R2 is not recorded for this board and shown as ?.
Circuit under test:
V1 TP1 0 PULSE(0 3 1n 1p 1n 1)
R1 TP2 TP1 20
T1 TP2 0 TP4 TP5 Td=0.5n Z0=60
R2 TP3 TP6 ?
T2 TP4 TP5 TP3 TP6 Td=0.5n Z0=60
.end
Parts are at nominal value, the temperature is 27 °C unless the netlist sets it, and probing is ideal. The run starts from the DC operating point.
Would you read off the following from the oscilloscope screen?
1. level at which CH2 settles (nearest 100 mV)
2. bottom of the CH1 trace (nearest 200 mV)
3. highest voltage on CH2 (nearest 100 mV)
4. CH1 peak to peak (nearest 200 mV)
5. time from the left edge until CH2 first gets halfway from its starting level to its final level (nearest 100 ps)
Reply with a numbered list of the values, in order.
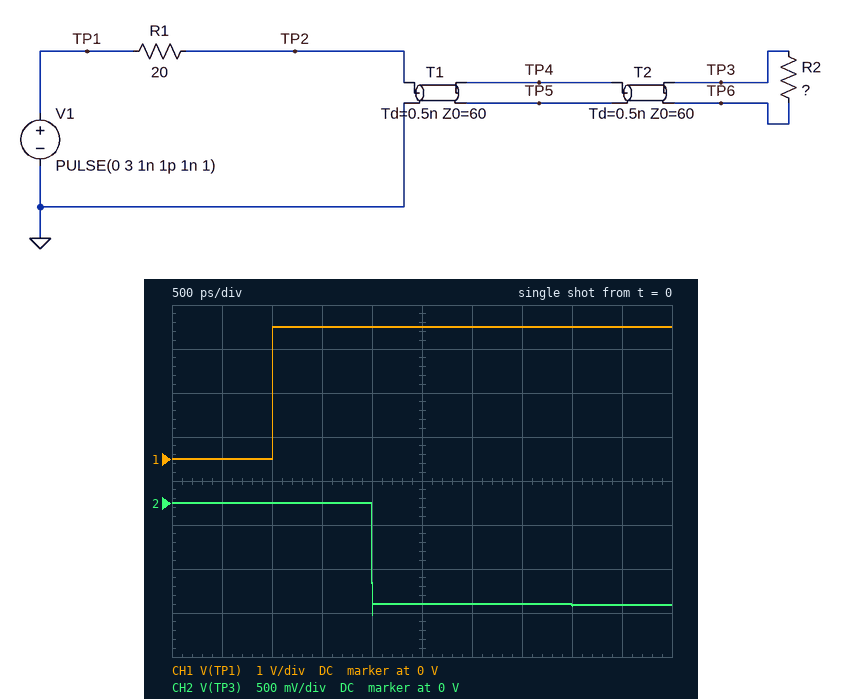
1. -1.2 V
2. 0 V
3. 0 V
4. 3.0 V
5. 2.0 ns
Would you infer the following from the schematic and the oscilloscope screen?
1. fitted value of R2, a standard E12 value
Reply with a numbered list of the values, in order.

1. 56 Ω
